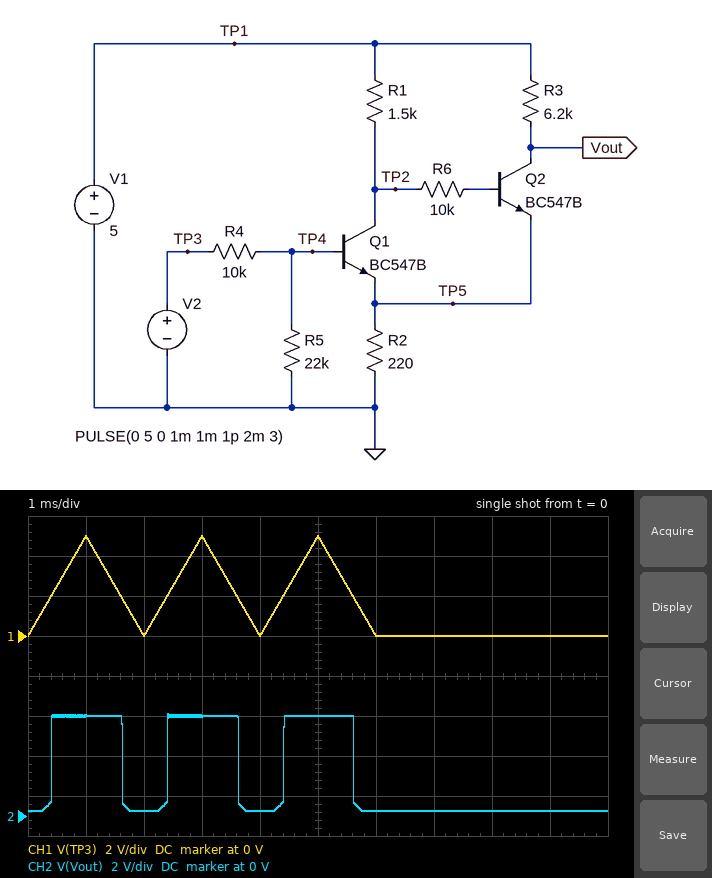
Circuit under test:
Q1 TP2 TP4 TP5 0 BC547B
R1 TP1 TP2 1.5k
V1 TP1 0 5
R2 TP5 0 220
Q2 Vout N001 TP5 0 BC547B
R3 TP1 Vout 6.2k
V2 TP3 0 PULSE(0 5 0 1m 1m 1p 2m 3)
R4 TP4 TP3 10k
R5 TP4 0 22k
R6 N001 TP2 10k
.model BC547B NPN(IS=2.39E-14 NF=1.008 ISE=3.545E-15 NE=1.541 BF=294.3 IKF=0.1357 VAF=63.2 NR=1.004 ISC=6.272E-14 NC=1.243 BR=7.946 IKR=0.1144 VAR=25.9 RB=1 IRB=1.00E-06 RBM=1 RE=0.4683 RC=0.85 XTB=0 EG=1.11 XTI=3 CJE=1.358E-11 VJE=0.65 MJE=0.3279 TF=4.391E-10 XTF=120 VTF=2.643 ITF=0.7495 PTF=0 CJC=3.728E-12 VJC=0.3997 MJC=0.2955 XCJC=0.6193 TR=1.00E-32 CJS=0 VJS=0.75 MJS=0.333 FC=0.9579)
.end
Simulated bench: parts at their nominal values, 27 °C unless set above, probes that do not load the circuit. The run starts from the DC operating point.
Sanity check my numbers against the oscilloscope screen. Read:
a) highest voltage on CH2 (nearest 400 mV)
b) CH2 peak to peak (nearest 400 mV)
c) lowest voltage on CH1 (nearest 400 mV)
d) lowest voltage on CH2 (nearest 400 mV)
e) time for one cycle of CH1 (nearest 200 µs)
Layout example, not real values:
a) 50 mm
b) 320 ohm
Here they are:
a) 5.2 V
b) 4.8 V
c) 0 V
d) 400 mV
e) 2.0 ms
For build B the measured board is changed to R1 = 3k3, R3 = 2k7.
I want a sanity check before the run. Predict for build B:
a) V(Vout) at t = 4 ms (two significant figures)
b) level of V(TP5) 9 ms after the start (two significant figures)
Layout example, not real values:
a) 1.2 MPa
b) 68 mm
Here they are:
a) 460 mV
b) 430 mV
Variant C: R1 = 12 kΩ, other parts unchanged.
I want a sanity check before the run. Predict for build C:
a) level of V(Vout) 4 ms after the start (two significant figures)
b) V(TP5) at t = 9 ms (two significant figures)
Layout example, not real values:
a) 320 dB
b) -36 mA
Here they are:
a) 230 mV
b) 210 mV
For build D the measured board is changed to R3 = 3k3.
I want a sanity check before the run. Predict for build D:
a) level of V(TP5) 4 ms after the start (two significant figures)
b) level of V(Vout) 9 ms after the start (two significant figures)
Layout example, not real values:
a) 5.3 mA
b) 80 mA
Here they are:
a) 380 mV
b) 400 mV
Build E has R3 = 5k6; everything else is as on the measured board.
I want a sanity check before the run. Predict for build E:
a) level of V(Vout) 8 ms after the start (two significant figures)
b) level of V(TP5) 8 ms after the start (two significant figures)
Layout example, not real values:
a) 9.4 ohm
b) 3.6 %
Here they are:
a) 280 mV
b) 260 mV
